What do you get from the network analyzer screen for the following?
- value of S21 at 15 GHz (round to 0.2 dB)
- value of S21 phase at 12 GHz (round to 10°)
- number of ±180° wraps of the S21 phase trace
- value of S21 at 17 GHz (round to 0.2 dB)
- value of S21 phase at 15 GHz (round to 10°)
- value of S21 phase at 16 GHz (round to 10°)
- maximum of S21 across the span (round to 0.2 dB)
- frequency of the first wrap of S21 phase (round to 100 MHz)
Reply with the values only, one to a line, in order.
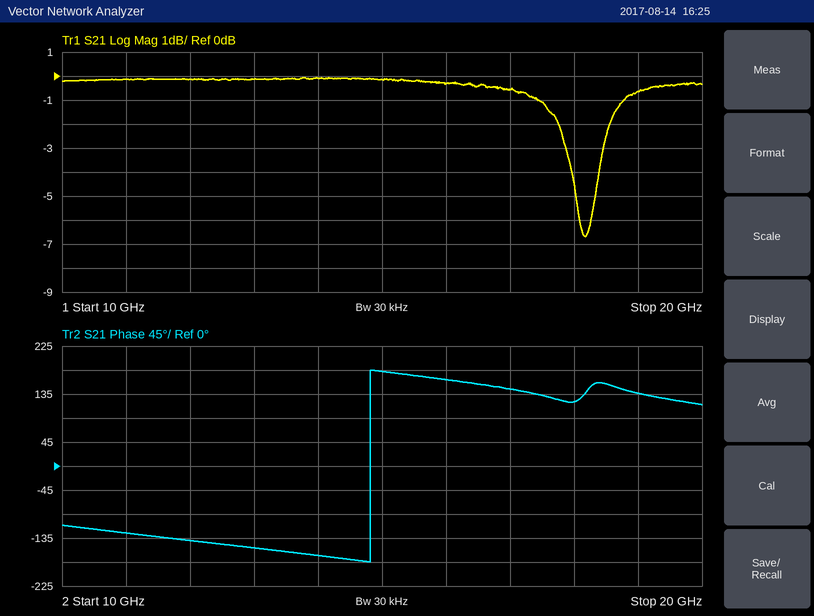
-0.2 dB
-140°
1
-0.6 dB
180°
160°
0.0 dB
14.8 GHz
